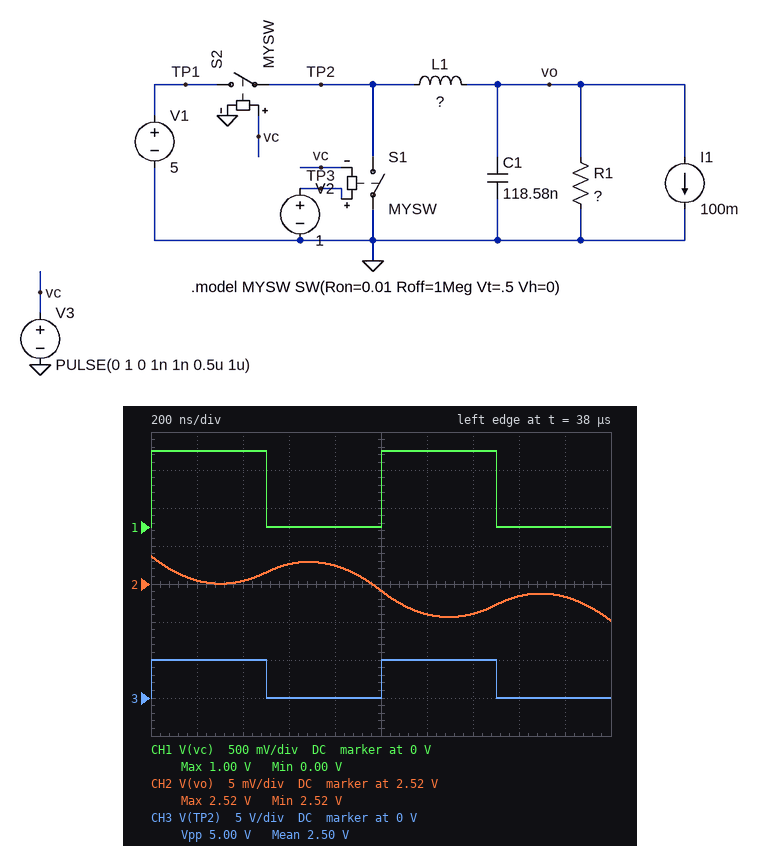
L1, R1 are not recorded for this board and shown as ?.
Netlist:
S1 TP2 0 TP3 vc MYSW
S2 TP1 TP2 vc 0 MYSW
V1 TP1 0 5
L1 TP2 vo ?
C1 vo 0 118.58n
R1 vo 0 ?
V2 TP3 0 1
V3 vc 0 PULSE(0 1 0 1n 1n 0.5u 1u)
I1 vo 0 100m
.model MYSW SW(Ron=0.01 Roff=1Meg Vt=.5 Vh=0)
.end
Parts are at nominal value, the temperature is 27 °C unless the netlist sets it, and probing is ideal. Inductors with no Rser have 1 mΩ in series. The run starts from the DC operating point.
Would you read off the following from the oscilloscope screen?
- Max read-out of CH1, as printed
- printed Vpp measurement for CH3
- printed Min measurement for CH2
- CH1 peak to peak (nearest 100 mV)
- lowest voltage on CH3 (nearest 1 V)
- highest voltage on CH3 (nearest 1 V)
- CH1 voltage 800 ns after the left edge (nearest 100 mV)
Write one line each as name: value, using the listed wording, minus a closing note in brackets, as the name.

Max read-out of CH1, as printed: 1.00 V
printed Vpp measurement for CH3: 5.00 V
printed Min measurement for CH2: 2.52 V
CH1 peak to peak: 1.0 V
lowest voltage on CH3: 0 V
highest voltage on CH3: 5 V
CH1 voltage 800 ns after the left edge: 0 V
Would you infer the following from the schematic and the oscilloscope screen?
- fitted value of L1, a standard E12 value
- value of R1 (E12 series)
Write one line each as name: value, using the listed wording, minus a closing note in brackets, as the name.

fitted value of L1, a standard E12 value: 270 µH
value of R1: 33 Ω
